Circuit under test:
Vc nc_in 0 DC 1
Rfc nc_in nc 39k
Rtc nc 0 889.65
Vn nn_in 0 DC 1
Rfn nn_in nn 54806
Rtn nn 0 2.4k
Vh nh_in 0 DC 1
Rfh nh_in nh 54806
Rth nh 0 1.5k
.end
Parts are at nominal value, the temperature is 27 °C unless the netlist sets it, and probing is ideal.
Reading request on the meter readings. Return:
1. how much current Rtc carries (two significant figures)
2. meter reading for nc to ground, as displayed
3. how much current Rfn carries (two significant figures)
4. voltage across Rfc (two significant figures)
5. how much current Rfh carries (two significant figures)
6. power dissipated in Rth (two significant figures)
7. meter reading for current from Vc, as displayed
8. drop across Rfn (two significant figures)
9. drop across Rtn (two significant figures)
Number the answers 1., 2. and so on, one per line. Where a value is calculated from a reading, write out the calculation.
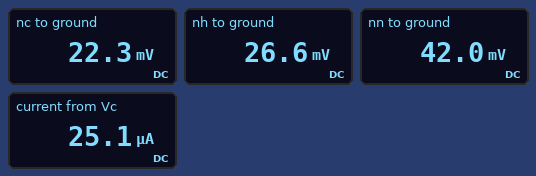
1. (22.3 mV) / 889.6 Ω = 25 µA
2. 22.3 mV
3. (1 V - 42 mV) / 54.81 kΩ = 17 µA
4. 1 V - 22.3 mV = 980 mV
5. (1 V - 26.6 mV) / 54.81 kΩ = 18 µA
6. (26.6 mV)^2 / 1.5 kΩ = 470 nW
7. 25.1 µA
8. 1 V - 42 mV = 960 mV
9. 42 mV = 42 mV
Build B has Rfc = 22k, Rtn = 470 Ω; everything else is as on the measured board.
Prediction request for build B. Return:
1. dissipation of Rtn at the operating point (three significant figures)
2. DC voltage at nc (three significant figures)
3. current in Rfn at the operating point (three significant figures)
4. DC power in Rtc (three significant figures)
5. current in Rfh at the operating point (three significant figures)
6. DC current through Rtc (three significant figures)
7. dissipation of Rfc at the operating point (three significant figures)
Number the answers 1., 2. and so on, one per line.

1. 154 nW
2. 38.9 mV
3. 18.1 µA
4. 1.70 µW
5. 17.8 µA
6. 43.7 µA
7. 42.0 µW
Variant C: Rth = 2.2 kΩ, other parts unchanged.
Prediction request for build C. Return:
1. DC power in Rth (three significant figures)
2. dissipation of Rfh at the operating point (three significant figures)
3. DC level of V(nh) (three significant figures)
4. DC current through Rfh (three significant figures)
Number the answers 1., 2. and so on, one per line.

1. 677 nW
2. 16.9 µW
3. 38.6 mV
4. 17.5 µA
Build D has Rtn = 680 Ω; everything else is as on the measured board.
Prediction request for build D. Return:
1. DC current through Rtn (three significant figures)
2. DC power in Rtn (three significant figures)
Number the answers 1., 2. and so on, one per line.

1. 18.0 µA
2. 221 nW
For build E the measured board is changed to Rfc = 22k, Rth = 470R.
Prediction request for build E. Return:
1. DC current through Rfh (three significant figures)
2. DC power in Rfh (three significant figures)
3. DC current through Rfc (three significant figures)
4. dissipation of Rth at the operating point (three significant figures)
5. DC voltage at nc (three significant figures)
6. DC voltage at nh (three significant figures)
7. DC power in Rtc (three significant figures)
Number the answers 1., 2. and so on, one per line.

1. 18.1 µA
2. 17.9 µW
3. 43.7 µA
4. 154 nW
5. 38.9 mV
6. 8.50 mV
7. 1.70 µW
